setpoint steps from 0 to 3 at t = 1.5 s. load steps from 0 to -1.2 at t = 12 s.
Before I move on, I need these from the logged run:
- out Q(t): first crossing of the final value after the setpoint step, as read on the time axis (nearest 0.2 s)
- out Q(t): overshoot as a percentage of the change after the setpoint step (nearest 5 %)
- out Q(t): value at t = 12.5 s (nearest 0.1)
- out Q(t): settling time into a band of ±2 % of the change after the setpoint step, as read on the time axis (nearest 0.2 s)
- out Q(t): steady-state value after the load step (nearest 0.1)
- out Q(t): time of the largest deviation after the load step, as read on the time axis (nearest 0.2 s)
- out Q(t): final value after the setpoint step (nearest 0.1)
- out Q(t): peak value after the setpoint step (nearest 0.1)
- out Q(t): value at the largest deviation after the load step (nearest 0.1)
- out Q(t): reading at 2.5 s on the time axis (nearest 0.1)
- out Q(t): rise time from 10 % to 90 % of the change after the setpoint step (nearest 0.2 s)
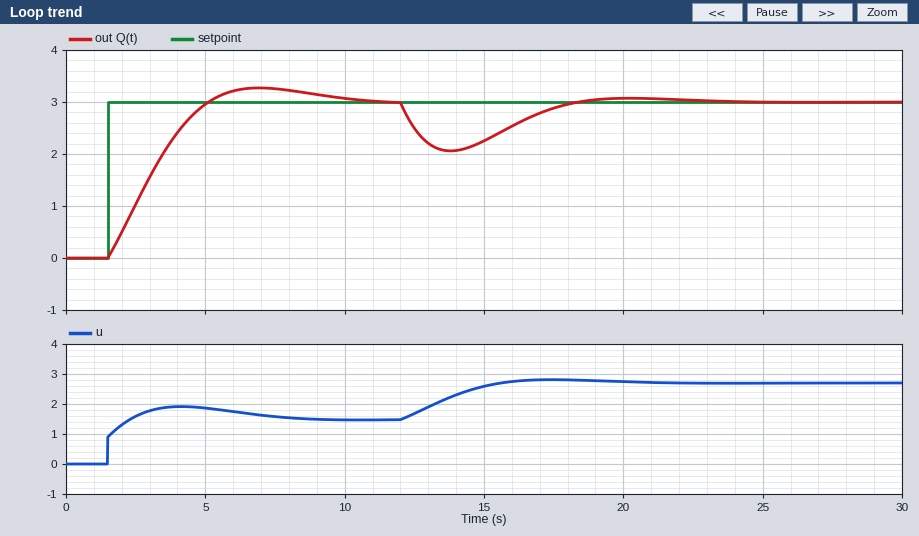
5.2 s
10 %
2.5
10.2 s
3.0
13.8 s
3.0
3.3
2.1
1.0
2.6 s
